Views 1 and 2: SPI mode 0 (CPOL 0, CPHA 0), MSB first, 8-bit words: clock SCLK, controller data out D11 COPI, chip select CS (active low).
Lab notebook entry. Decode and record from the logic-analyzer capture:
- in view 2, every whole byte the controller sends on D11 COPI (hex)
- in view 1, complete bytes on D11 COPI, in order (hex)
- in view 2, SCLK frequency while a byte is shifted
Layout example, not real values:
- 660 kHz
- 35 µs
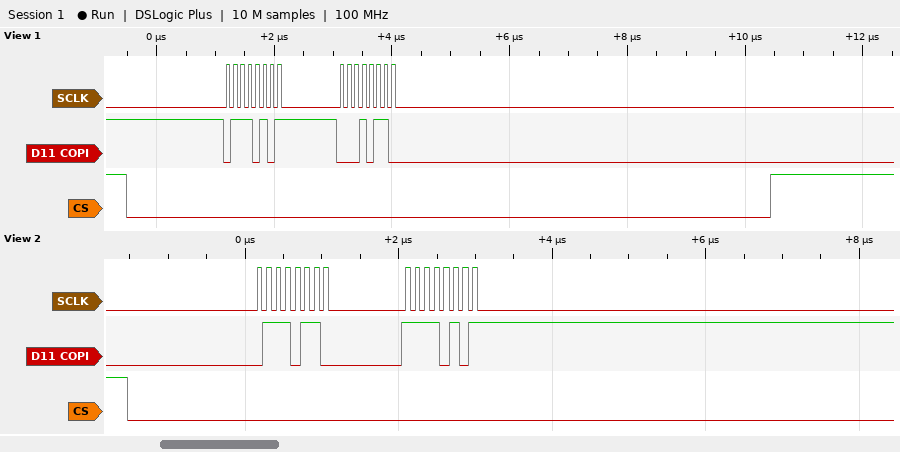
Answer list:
- 0x76 0xF5
- 75 16
- 8 MHz
